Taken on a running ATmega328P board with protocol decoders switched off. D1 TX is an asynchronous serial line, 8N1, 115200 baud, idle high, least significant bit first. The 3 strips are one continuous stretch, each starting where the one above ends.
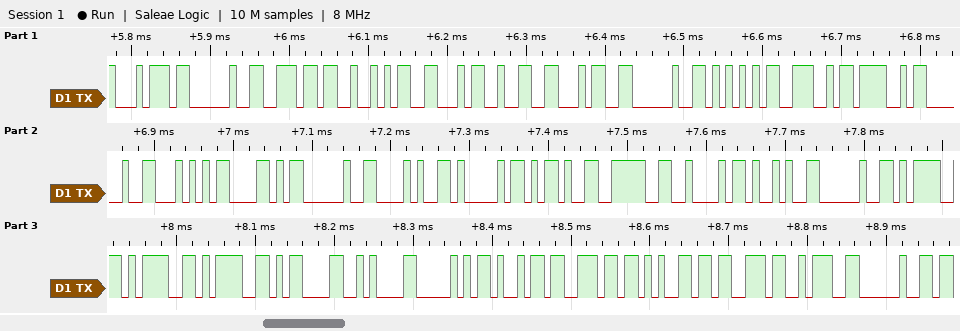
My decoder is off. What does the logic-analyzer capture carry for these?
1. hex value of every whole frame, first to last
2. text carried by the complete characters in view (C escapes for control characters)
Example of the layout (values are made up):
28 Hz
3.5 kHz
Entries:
0x74 0x20 0x6E 0x52 0x46 0x32 0x34 0x20 0x55 0x4E 0x4F 0x20 0x54 0x58 0x20 0x28 0x41 0x2D 0x3E 0x42 0x29 0x20 0x3D 0x3D 0x3D 0x0D 0x0A 0x50 0x69 0x6E 0x65 0x73 0x3A 0x20
"t nRF24 UNO TX (A->B) ===\r\nPines: "
